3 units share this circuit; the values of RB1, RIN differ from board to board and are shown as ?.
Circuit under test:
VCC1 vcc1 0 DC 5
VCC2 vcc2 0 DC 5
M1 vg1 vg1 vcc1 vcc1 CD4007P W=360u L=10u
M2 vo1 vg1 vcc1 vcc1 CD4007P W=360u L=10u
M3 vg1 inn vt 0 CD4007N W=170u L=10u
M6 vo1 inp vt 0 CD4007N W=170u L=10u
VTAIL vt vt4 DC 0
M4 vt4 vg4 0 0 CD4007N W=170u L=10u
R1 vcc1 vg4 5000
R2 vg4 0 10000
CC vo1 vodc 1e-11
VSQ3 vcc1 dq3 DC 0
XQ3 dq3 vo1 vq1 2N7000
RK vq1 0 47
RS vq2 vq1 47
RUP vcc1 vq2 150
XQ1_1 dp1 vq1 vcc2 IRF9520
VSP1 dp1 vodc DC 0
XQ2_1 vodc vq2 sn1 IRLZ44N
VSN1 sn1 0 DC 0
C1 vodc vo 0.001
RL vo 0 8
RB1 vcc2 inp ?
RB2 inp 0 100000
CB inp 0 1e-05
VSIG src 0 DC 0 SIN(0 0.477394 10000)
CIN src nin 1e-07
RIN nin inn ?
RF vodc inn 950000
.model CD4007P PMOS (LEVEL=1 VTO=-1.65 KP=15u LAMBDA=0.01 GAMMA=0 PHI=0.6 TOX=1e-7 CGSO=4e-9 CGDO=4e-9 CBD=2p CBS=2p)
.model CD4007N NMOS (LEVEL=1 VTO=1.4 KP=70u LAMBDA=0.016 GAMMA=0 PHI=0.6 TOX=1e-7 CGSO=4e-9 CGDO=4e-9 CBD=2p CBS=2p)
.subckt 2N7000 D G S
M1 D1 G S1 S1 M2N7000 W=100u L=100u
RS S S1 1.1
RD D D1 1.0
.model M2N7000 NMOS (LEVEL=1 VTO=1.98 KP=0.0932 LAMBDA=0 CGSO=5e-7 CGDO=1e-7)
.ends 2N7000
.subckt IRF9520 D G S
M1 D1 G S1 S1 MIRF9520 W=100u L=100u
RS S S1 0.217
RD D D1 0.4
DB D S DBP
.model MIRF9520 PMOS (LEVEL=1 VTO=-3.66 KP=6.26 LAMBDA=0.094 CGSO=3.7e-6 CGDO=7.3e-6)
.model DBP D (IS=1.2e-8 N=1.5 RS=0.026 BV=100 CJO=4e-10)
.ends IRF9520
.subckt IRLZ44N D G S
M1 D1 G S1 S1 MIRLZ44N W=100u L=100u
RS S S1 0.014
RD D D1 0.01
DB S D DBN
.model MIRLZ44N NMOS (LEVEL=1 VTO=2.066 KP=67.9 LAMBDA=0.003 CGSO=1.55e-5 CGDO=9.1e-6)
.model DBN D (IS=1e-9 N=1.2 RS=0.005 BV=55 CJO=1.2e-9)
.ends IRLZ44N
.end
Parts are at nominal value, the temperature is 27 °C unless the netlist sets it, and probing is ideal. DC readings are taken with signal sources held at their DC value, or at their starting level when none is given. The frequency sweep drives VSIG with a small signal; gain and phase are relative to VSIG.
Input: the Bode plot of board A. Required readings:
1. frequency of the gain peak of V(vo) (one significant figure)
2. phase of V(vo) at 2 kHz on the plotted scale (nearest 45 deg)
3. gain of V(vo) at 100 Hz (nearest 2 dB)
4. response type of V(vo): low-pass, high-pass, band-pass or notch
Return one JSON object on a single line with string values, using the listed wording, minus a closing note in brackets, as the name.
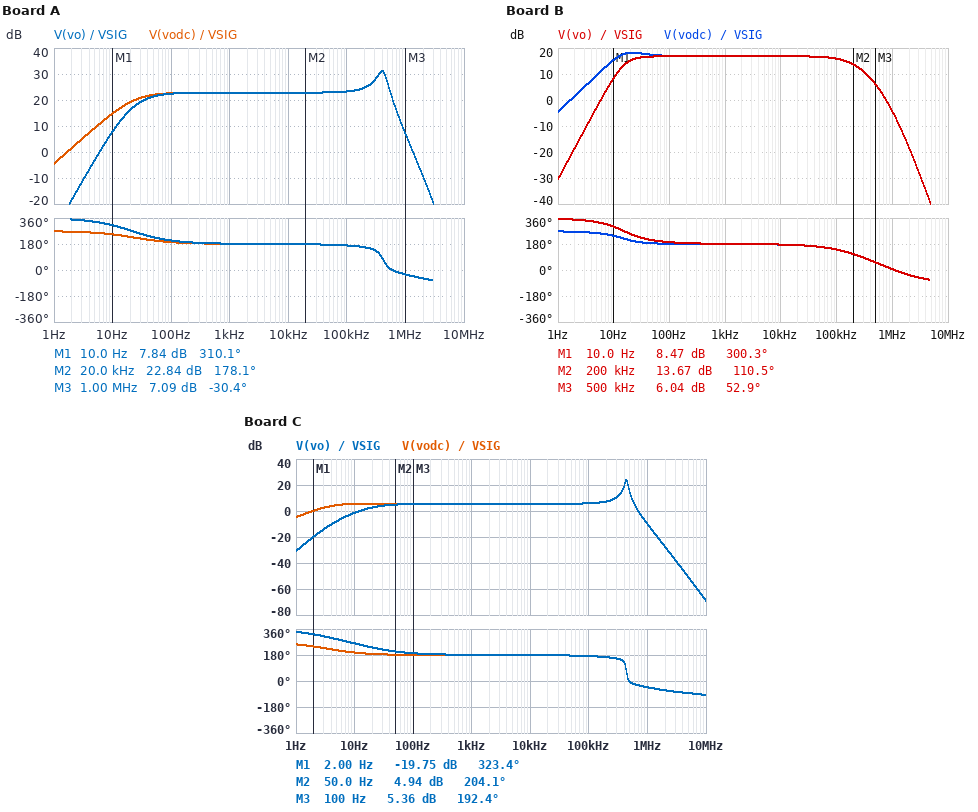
{"frequency of the gain peak of V(vo)": "400 kHz", "phase of V(vo) at 2 kHz on the plotted scale": "180 deg", "gain of V(vo) at 100 Hz": "22 dB", "response type of V(vo): low-pass, high-pass, band-pass or notch": "band-pass"}
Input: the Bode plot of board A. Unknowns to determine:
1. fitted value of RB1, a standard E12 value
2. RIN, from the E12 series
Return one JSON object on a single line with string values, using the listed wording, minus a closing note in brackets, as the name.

{"fitted value of RB1, a standard E12 value": "120 kΩ", "RIN, from the E12 series": "68 kΩ"}
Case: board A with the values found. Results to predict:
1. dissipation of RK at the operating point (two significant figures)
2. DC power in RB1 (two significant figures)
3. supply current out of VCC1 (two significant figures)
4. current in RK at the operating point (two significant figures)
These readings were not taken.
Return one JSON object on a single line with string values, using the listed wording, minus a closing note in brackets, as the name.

{"dissipation of RK at the operating point": "31 mW", "DC power in RB1": "62 µW", "supply current out of VCC1": "26 mA", "current in RK at the operating point": "26 mA"}
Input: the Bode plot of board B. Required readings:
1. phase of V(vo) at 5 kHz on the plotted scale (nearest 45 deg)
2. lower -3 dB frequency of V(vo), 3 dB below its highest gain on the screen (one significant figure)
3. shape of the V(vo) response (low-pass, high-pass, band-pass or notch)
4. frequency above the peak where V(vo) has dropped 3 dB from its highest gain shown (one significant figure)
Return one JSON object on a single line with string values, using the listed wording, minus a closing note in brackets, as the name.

{"phase of V(vo) at 5 kHz on the plotted scale": "180 deg", "lower -3 dB frequency of V(vo), 3 dB below its highest gain on the screen": "20 Hz", "shape of the V(vo) response": "band-pass", "frequency above the peak where V(vo) has dropped 3 dB from its highest gain shown": "200 kHz"}
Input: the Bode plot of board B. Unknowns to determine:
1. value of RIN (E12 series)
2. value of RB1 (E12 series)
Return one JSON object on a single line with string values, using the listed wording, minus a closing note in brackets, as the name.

{"value of RIN": "68 kΩ", "value of RB1": "39 kΩ"}
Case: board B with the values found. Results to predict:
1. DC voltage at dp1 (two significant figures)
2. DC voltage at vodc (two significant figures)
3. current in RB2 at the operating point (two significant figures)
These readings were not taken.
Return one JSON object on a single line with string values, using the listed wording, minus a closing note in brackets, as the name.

{"DC voltage at dp1": "4.1 V", "DC voltage at vodc": "4.1 V", "current in RB2 at the operating point": "36 µA"}
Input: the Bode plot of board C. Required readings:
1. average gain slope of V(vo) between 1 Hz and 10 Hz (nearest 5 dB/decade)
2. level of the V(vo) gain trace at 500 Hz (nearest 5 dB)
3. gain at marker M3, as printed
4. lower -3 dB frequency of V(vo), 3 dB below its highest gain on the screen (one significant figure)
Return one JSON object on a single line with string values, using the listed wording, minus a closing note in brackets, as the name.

{"average gain slope of V(vo) between 1 Hz and 10 Hz": "30 dB/decade", "level of the V(vo) gain trace at 500 Hz": "5 dB", "gain at marker M3, as printed": "5.36 dB", "lower -3 dB frequency of V(vo), 3 dB below its highest gain on the screen": "400 kHz"}
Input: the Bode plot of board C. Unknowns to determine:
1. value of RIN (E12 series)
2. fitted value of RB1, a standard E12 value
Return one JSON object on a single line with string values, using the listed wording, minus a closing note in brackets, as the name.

{"value of RIN": "470 kΩ", "fitted value of RB1, a standard E12 value": "47 kΩ"}
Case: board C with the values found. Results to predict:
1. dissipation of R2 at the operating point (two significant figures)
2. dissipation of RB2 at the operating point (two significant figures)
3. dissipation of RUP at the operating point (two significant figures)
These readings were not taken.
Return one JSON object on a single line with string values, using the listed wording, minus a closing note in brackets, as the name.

{"dissipation of R2 at the operating point": "1.1 mW", "dissipation of RB2 at the operating point": "120 µW", "dissipation of RUP at the operating point": "56 mW"}
